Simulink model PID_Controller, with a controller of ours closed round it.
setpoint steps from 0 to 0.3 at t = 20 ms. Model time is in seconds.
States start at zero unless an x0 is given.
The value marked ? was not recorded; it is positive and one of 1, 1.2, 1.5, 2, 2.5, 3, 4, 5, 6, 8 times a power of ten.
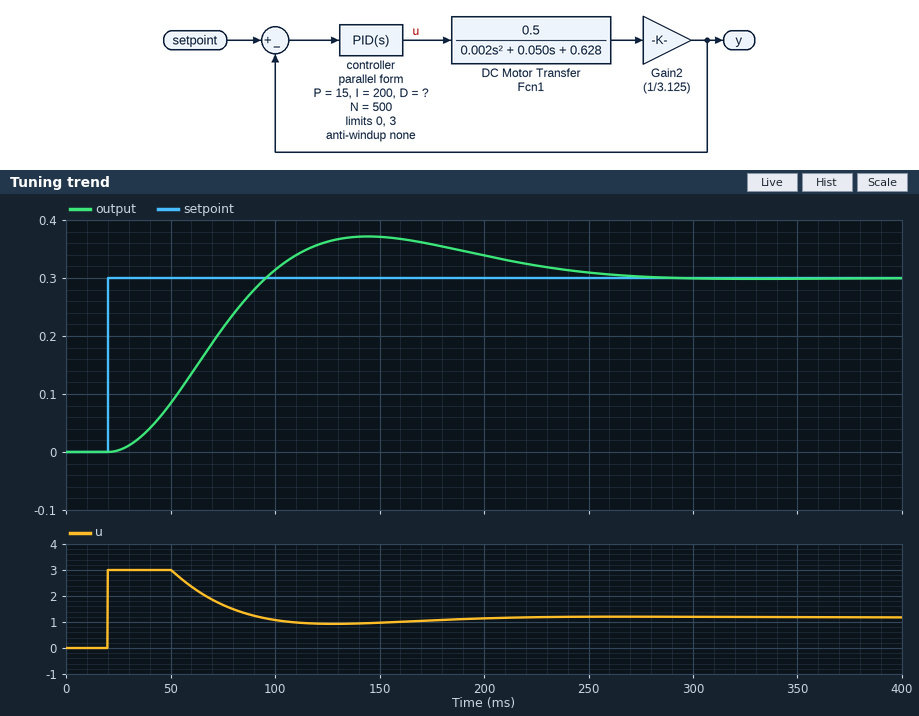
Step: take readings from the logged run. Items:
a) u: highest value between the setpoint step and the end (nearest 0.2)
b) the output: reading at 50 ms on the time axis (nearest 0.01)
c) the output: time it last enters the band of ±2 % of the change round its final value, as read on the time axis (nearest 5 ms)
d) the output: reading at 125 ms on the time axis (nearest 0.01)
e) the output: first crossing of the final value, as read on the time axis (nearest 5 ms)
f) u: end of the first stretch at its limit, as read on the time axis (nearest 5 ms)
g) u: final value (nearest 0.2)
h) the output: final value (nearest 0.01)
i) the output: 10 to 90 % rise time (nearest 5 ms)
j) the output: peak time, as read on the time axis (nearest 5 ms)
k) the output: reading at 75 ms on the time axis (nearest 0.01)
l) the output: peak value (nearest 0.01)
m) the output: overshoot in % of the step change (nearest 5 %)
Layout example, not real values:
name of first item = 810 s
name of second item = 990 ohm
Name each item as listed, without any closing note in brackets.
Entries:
u: highest value between the setpoint step and the end = 3.0
the output: reading at 50 ms on the time axis = 0.08
the output: time it last enters the band of ±2 % of the change round its final value, as read on the time axis = 260 ms
the output: reading at 125 ms on the time axis = 0.36
the output: first crossing of the final value, as read on the time axis = 95 ms
u: end of the first stretch at its limit, as read on the time axis = 50 ms
u: final value = 1.2
the output: final value = 0.30
the output: 10 to 90 % rise time = 50 ms
the output: peak time, as read on the time axis = 145 ms
the output: reading at 75 ms on the time axis = 0.21
the output: peak value = 0.37
the output: overshoot in % of the step change = 25 %
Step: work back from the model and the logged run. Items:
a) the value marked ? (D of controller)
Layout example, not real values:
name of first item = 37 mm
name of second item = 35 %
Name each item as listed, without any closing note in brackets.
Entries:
the value marked ? = 0.4
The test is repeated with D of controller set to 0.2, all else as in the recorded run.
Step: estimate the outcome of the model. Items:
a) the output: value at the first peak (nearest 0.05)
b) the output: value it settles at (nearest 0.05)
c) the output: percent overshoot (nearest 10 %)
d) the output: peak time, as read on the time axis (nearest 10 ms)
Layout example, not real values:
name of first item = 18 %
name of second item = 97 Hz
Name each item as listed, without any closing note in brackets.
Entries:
the output: value at the first peak = 0.40
the output: value it settles at = 0.30
the output: percent overshoot = 30 %
the output: peak time, as read on the time axis = 130 ms
